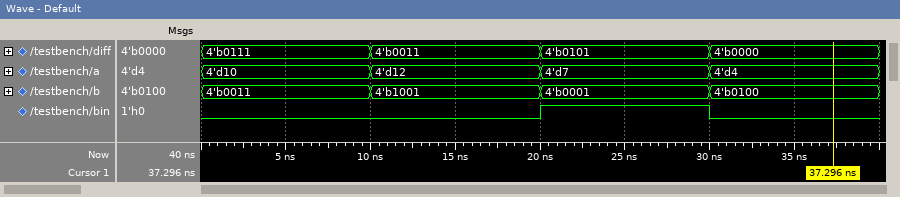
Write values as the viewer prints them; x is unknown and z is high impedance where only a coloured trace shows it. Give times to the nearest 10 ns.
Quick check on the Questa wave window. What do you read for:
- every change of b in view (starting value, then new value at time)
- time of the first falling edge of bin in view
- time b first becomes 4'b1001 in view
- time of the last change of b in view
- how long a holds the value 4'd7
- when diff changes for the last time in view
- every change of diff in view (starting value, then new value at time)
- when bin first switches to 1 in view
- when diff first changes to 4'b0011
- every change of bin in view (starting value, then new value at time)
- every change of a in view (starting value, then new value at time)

4'b0011, 4'b1001 at 10 ns, 4'b0001 at 20 ns, 4'b0100 at 30 ns
30 ns
10 ns
30 ns
10 ns
30 ns
4'b0111, 4'b0011 at 10 ns, 4'b0101 at 20 ns, 4'b0000 at 30 ns
20 ns
10 ns
0, 1 at 20 ns, 0 at 30 ns
4'd10, 4'd12 at 10 ns, 4'd7 at 20 ns, 4'd4 at 30 ns
